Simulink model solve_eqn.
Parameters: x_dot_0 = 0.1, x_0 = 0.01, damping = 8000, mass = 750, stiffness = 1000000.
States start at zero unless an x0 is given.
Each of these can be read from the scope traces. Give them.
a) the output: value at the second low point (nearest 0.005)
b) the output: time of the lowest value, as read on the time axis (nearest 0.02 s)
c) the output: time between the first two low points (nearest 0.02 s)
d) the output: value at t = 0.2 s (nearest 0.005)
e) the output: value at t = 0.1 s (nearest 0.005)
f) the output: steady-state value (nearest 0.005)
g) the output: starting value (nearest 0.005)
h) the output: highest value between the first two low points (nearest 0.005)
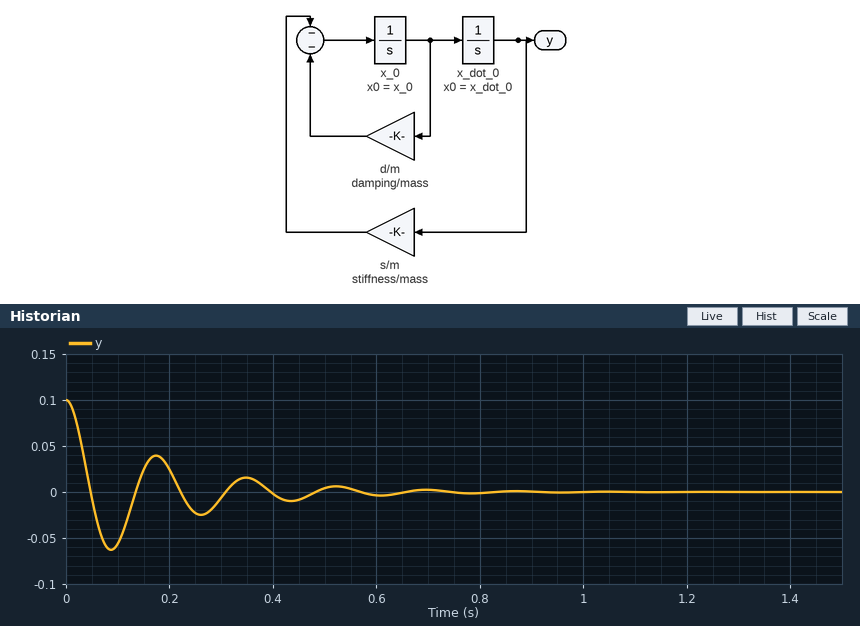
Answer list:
-0.025
0.08 s
0.18 s
0.025
-0.055
0.000
0.100
0.040
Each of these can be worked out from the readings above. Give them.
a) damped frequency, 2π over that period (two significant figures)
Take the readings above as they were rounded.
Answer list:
35 rad/s
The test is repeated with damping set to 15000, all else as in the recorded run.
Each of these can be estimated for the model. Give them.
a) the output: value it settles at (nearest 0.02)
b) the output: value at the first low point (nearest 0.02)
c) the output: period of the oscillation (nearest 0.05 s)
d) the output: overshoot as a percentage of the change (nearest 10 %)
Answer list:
0.00
-0.04
0.20 s
40 %
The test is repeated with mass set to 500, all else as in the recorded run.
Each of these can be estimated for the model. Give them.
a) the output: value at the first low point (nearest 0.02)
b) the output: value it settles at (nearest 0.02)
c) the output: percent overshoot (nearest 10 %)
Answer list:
-0.06
0.00
60 %
